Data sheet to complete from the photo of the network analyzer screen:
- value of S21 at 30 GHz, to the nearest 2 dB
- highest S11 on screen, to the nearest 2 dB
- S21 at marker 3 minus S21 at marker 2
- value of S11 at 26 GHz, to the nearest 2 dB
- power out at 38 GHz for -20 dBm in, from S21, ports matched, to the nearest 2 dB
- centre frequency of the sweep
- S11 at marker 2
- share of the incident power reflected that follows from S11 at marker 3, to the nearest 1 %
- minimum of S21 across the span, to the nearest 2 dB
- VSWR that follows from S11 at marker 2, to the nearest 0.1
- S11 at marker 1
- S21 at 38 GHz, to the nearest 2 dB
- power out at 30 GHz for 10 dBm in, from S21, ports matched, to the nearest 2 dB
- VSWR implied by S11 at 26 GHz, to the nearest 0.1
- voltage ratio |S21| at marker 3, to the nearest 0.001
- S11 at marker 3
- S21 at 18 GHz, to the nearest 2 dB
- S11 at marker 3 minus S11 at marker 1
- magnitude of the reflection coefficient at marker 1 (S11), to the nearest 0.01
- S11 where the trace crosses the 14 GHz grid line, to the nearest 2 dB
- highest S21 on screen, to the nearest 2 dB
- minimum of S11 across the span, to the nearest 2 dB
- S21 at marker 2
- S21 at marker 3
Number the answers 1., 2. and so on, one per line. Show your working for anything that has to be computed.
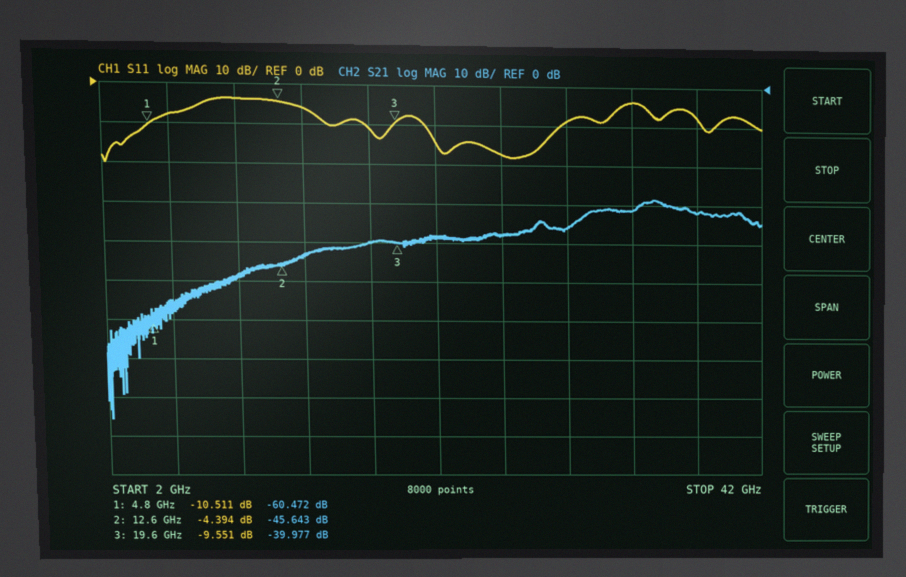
1. -36 dB
2. -4 dB
3. -39.977 − (-45.643) = 5.666 dB
4. -18 dB
5. -20 dBm + (-32 dB) = -52 dBm
6. 22 GHz
7. -4.394 dB
8. 10^(-9.551/10) ≈ 11 %
9. -86 dB
10. (1 + 0.6030)/(1 − 0.6030) ≈ 4.0
11. -10.511 dB
12. -32 dB
13. 10 dBm + (-36 dB) = -26 dBm
14. |Γ| = 10^(-18/20) = 0.1259; VSWR = (1 + 0.1259)/(1 − 0.1259) ≈ 1.3
15. 10^(-39.977/20) ≈ 0.010
16. -9.551 dB
17. -40 dB
18. -9.551 − (-10.511) = 0.960 dB
19. 10^(-10.511/20) ≈ 0.30
20. -6 dB
21. -28 dB
22. -20 dB
23. -45.643 dB
24. -39.977 dB
